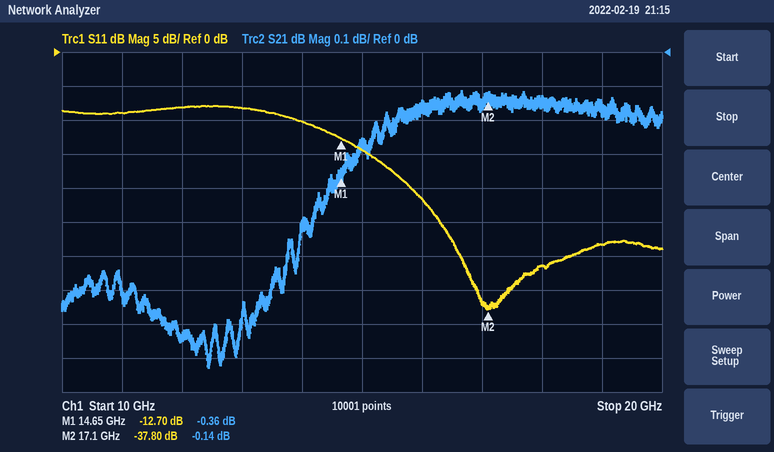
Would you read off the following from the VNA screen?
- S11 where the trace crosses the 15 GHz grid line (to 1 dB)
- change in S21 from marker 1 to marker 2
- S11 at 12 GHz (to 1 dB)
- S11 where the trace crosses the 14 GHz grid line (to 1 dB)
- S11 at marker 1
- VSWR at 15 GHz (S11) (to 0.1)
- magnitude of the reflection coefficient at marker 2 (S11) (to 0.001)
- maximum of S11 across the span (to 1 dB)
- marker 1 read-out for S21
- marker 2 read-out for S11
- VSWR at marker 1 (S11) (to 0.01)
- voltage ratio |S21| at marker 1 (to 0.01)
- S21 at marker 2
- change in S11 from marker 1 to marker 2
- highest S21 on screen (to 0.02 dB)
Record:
-14 dB
0.22 dB
-8 dB
-10 dB
-12.70 dB
1.5
0.013
-8 dB
-0.36 dB
-37.80 dB
1.60
0.96
-0.14 dB
-25.10 dB
-0.12 dB
